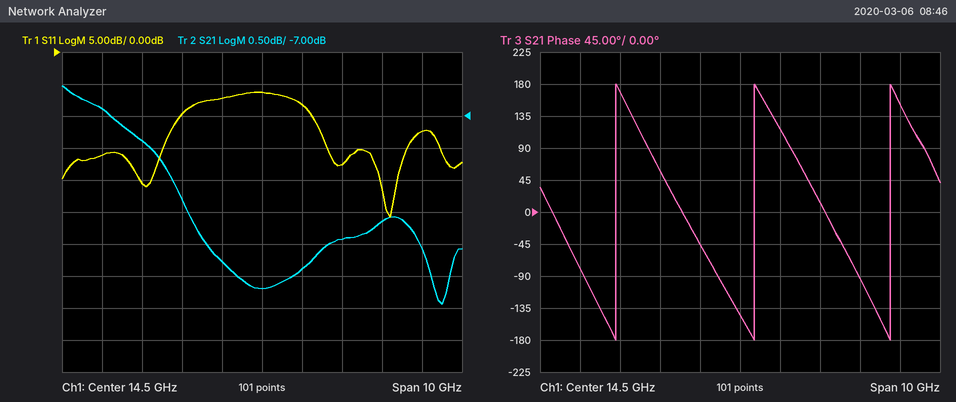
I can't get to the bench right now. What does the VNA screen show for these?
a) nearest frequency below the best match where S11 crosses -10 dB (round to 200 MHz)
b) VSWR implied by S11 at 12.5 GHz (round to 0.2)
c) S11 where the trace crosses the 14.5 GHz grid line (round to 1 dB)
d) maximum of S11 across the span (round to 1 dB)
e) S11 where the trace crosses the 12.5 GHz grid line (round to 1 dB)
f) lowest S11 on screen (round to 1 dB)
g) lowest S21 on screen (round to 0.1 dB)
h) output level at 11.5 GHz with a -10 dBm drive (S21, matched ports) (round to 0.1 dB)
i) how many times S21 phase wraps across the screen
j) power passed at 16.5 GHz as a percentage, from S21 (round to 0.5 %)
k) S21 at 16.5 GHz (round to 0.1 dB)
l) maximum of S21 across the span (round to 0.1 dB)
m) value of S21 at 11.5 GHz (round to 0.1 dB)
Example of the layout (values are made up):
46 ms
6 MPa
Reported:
15.8 GHz
2.0
-6 dB
-6 dB
-10 dB
-26 dB
-9.9 dB
-17.4 dBm
3
13.0 %
-8.9 dB
-6.5 dB
-7.4 dB
